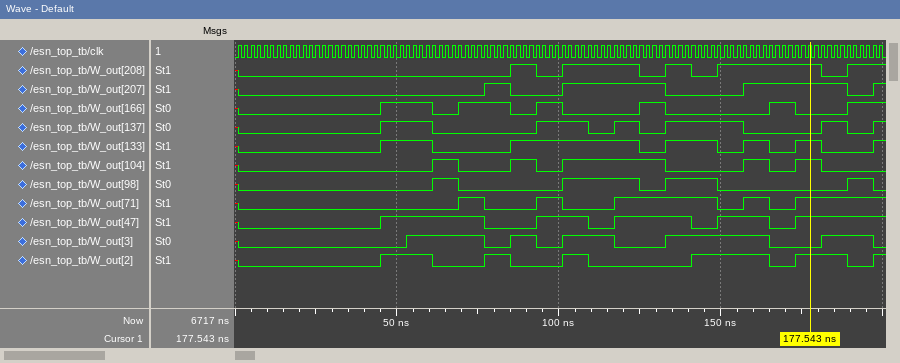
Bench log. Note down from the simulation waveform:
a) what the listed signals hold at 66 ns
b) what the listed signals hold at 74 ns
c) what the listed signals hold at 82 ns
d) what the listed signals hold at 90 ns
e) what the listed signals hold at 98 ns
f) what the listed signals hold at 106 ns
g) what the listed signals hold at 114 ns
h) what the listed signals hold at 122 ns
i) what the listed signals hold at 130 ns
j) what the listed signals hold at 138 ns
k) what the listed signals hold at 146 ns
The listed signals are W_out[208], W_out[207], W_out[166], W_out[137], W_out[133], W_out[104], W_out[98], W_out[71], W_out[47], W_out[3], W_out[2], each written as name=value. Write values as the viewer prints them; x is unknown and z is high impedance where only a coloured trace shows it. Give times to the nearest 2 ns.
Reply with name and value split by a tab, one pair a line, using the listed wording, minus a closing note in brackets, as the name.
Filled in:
what the listed signals hold at 66 ns	W_out[208]=0, W_out[207]=0, W_out[166]=0, W_out[137]=0, W_out[133]=0, W_out[104]=1, W_out[98]=1, W_out[71]=0, W_out[47]=1, W_out[3]=1, W_out[2]=0
what the listed signals hold at 74 ns	W_out[208]=0, W_out[207]=0, W_out[166]=1, W_out[137]=0, W_out[133]=0, W_out[104]=0, W_out[98]=0, W_out[71]=1, W_out[47]=1, W_out[3]=1, W_out[2]=0
what the listed signals hold at 82 ns	W_out[208]=0, W_out[207]=1, W_out[166]=1, W_out[137]=0, W_out[133]=0, W_out[104]=0, W_out[98]=0, W_out[71]=0, W_out[47]=0, W_out[3]=0, W_out[2]=1
what the listed signals hold at 90 ns	W_out[208]=1, W_out[207]=0, W_out[166]=0, W_out[137]=0, W_out[133]=1, W_out[104]=1, W_out[98]=0, W_out[71]=0, W_out[47]=0, W_out[3]=1, W_out[2]=0
what the listed signals hold at 98 ns	W_out[208]=0, W_out[207]=0, W_out[166]=1, W_out[137]=1, W_out[133]=1, W_out[104]=0, W_out[98]=0, W_out[71]=1, W_out[47]=1, W_out[3]=0, W_out[2]=0
what the listed signals hold at 106 ns	W_out[208]=1, W_out[207]=1, W_out[166]=0, W_out[137]=1, W_out[133]=1, W_out[104]=1, W_out[98]=1, W_out[71]=0, W_out[47]=1, W_out[3]=1, W_out[2]=1
what the listed signals hold at 114 ns	W_out[208]=1, W_out[207]=1, W_out[166]=0, W_out[137]=0, W_out[133]=1, W_out[104]=1, W_out[98]=1, W_out[71]=0, W_out[47]=0, W_out[3]=1, W_out[2]=0
what the listed signals hold at 122 ns	W_out[208]=1, W_out[207]=1, W_out[166]=0, W_out[137]=1, W_out[133]=1, W_out[104]=1, W_out[98]=1, W_out[71]=1, W_out[47]=1, W_out[3]=0, W_out[2]=0
what the listed signals hold at 130 ns	W_out[208]=0, W_out[207]=1, W_out[166]=1, W_out[137]=0, W_out[133]=0, W_out[104]=1, W_out[98]=0, W_out[71]=1, W_out[47]=1, W_out[3]=0, W_out[2]=0
what the listed signals hold at 138 ns	W_out[208]=1, W_out[207]=0, W_out[166]=0, W_out[137]=1, W_out[133]=1, W_out[104]=0, W_out[98]=1, W_out[71]=1, W_out[47]=1, W_out[3]=1, W_out[2]=0
what the listed signals hold at 146 ns	W_out[208]=0, W_out[207]=0, W_out[166]=0, W_out[137]=1, W_out[133]=1, W_out[104]=0, W_out[98]=1, W_out[71]=1, W_out[47]=0, W_out[3]=1, W_out[2]=1
